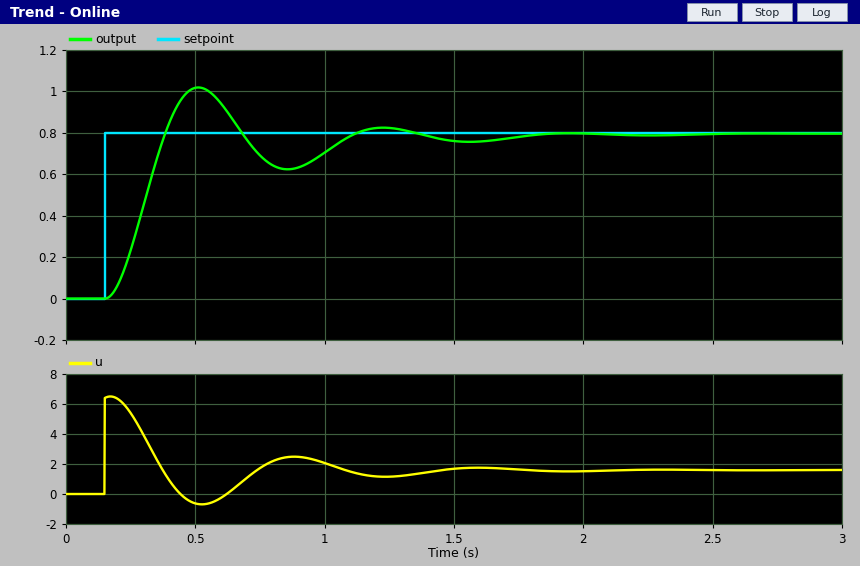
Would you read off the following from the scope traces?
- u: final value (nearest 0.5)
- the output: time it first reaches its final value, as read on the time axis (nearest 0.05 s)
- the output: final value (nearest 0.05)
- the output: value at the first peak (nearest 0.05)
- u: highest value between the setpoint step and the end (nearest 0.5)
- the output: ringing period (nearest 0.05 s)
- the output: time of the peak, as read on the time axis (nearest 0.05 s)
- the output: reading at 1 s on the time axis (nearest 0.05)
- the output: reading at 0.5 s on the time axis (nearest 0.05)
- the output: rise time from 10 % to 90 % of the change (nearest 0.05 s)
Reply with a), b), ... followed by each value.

a) 1.5
b) 0.40 s
c) 0.80
d) 1.00
e) 6.5
f) 0.70 s
g) 0.50 s
h) 0.70
i) 1.00
j) 0.15 s
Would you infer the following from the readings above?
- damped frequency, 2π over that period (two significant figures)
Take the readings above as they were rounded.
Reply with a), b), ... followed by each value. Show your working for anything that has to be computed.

a) 2π / 0.7 = 9.0 rad/s
